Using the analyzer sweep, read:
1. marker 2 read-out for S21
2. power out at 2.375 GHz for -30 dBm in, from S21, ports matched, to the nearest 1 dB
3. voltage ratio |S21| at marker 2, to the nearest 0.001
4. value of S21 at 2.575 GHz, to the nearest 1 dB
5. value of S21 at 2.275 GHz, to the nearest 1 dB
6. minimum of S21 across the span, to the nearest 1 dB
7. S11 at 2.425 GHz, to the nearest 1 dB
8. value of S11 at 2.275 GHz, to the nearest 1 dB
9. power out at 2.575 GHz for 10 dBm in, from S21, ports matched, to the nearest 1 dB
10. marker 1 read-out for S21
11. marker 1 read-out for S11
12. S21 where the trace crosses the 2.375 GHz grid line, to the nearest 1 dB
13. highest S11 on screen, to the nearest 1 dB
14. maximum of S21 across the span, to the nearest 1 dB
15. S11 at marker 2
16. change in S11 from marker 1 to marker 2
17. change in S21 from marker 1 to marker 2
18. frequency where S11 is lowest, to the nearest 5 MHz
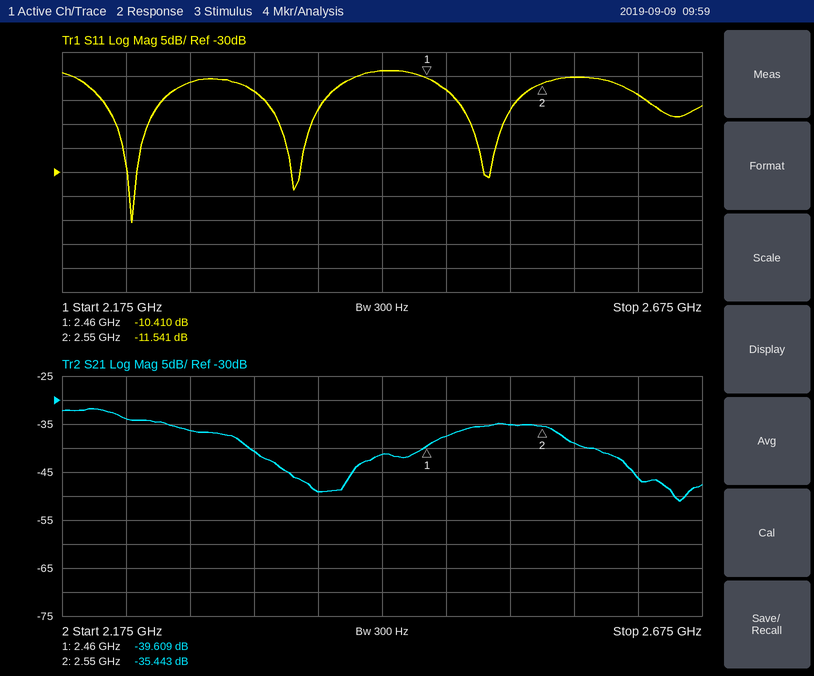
-35.443 dB
-79 dBm
0.017
-39 dB
-36 dB
-51 dB
-9 dB
-11 dB
-29 dBm
-39.609 dB
-10.410 dB
-49 dB
-9 dB
-32 dB
-11.541 dB
-1.131 dB
4.166 dB
2.230 GHz
